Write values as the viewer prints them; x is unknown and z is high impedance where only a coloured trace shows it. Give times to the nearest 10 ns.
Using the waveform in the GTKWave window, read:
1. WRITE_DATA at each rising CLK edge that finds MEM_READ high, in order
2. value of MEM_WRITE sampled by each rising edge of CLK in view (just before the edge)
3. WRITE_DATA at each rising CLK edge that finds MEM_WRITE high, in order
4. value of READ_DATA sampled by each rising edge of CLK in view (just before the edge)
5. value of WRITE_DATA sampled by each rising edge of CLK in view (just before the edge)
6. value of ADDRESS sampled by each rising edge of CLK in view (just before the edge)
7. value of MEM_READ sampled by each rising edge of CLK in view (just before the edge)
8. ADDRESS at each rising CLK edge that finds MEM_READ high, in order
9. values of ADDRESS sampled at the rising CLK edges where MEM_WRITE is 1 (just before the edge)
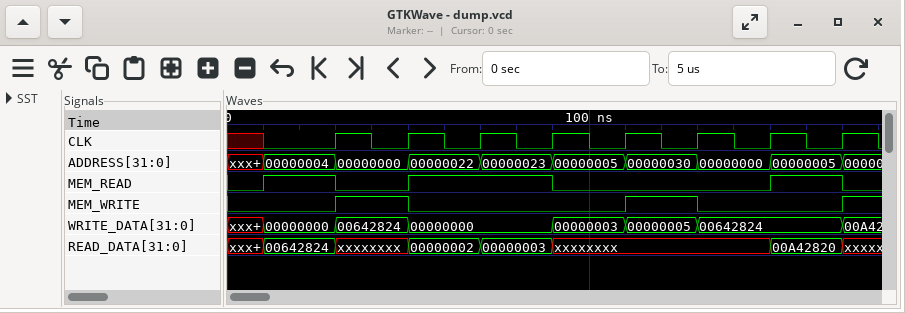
00000000, 00000000, 00000000, 00642824
0 1 0 0 0 1 0 0
00642824, 00000005
00642824, xxxxxxxx, 00000002, 00000003, xxxxxxxx, xxxxxxxx, xxxxxxxx, 00A42820
00000000, 00642824, 00000000, 00000000, 00000003, 00000005, 00642824, 00642824
00000004, 00000000, 00000022, 00000023, 00000005, 00000030, 00000000, 00000005
1 0 1 1 0 0 0 1
00000004, 00000022, 00000023, 00000005
00000000, 00000030
